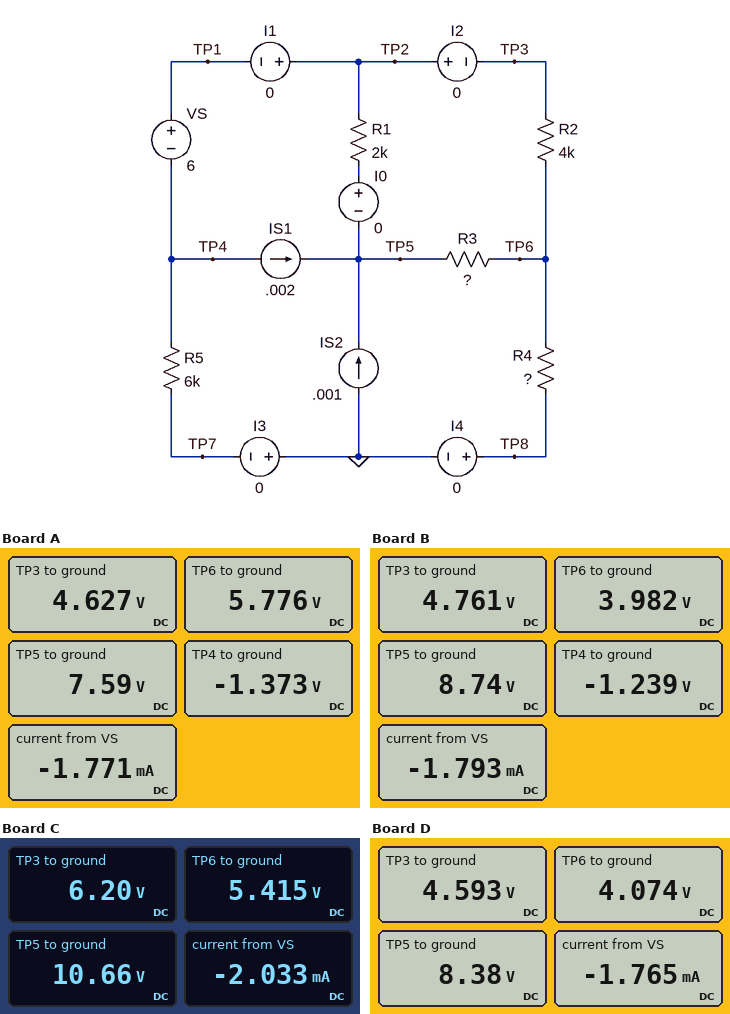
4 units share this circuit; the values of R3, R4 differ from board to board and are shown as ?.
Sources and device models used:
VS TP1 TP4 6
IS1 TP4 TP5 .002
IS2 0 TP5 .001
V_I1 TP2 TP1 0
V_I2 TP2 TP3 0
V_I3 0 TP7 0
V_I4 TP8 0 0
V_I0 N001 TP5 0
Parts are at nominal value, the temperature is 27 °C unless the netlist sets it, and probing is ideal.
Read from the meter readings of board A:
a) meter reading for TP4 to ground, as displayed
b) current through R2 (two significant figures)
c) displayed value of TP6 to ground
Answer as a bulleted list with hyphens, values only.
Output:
- -1.373 V
- 290 µA
- 5.776 V
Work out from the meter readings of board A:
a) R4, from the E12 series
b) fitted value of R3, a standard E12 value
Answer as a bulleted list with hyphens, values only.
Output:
- 4.7 kΩ
- 1.2 kΩ
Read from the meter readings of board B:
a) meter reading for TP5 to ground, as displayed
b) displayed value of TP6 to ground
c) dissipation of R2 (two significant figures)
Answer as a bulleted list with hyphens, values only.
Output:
- 8.74 V
- 3.982 V
- 150 µW
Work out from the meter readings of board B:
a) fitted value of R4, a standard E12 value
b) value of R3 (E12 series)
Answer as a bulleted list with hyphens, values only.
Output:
- 3.3 kΩ
- 4.7 kΩ
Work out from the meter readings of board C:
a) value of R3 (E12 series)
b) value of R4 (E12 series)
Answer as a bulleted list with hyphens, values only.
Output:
- 6.8 kΩ
- 5.6 kΩ
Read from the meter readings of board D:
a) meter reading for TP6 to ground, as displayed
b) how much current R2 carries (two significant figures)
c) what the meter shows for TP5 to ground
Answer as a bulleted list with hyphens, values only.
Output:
- 4.074 V
- 130 µA
- 8.38 V
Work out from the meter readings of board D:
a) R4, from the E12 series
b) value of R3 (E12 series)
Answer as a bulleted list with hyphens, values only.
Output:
- 3.3 kΩ
- 3.9 kΩ
